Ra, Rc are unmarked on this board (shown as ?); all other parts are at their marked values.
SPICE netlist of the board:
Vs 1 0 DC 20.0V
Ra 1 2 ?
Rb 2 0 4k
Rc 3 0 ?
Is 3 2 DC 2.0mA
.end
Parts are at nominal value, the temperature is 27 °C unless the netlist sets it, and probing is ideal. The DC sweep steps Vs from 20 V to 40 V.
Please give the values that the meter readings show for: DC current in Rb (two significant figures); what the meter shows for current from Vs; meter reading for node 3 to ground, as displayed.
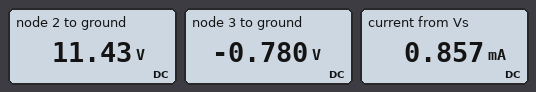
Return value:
2.9 mA
0.857 mA
-0.780 V
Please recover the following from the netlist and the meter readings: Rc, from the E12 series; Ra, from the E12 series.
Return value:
390 Ω
10 kΩ
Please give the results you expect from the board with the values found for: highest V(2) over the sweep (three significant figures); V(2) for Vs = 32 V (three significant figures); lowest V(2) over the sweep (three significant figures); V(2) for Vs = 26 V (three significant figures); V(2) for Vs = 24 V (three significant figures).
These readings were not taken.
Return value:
17.1 V
14.9 V
11.4 V
13.1 V
12.6 V
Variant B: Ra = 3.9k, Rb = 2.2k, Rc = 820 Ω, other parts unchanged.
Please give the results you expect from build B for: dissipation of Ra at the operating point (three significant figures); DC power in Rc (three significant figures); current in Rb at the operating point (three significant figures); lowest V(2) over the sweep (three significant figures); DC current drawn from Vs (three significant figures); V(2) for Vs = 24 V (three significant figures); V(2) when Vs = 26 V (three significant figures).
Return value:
25.5 mW
3.28 mW
4.56 mA
10.0 V
2.56 mA
11.5 V
12.2 V
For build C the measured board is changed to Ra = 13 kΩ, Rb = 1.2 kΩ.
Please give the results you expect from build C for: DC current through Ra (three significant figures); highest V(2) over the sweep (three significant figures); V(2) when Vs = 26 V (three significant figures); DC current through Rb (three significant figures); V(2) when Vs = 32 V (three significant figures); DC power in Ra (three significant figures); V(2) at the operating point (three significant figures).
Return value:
1.24 mA
5.58 V
4.39 V
3.24 mA
4.90 V
20.0 mW
3.89 V
